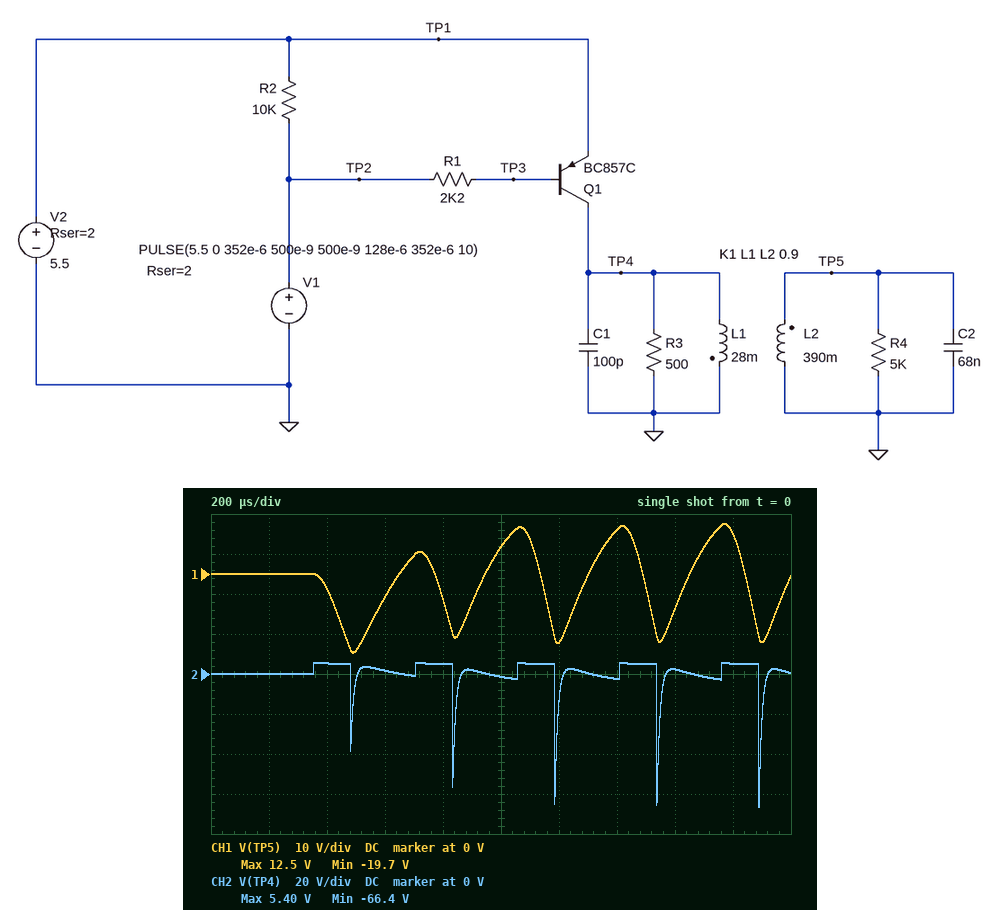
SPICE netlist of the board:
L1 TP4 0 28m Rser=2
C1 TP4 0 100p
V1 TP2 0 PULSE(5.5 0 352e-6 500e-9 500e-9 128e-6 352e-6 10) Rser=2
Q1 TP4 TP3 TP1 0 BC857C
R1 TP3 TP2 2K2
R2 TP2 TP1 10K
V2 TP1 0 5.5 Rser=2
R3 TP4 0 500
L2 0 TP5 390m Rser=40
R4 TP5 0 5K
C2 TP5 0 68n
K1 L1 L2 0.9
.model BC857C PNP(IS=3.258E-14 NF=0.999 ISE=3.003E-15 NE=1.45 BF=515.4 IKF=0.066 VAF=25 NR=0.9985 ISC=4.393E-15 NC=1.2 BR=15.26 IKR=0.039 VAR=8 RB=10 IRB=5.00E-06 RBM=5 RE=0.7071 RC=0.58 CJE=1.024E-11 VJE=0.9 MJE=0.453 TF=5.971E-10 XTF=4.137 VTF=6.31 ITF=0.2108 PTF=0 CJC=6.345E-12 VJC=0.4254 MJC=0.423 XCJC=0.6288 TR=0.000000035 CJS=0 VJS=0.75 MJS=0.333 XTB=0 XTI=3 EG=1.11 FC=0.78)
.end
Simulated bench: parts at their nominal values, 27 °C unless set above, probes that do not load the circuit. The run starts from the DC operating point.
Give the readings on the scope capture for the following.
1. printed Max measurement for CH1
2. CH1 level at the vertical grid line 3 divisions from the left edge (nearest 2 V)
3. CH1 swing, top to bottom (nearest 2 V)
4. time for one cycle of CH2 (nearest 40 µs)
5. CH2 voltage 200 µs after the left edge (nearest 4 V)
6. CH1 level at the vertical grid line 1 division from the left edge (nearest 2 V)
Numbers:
12.5 V
-6 V
32 V
360 µs
0 V
0 V
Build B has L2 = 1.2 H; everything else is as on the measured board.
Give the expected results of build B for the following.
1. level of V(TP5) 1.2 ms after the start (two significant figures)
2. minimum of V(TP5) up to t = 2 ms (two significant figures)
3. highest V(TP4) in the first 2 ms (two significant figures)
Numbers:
-8.5 V
-14 V
5.4 V
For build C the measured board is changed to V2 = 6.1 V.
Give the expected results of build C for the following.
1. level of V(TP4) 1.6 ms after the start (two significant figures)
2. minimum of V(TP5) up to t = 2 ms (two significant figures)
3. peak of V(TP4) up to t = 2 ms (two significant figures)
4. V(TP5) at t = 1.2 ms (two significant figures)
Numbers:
2.5 V
-22 V
6.0 V
-19 V
